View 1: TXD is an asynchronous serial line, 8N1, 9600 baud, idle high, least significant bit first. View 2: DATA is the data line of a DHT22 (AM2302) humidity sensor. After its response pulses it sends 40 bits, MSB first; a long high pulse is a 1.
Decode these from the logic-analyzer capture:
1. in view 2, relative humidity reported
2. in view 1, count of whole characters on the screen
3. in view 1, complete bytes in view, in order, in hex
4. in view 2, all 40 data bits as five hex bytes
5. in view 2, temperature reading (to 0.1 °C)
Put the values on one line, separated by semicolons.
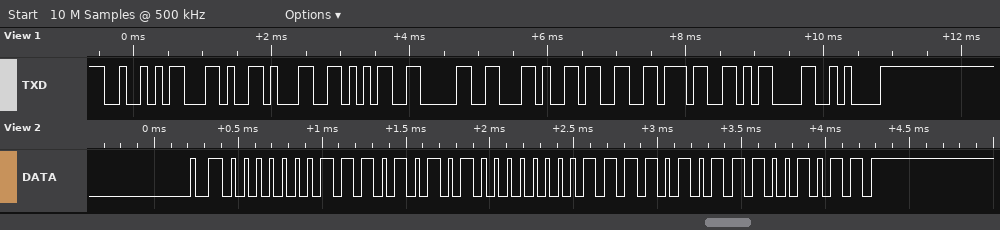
46.9 %; 10; 52 2C 31 35 30 2C 33 37 0D 0A; 01 D5 00 F5 CB; 24.5 °C
